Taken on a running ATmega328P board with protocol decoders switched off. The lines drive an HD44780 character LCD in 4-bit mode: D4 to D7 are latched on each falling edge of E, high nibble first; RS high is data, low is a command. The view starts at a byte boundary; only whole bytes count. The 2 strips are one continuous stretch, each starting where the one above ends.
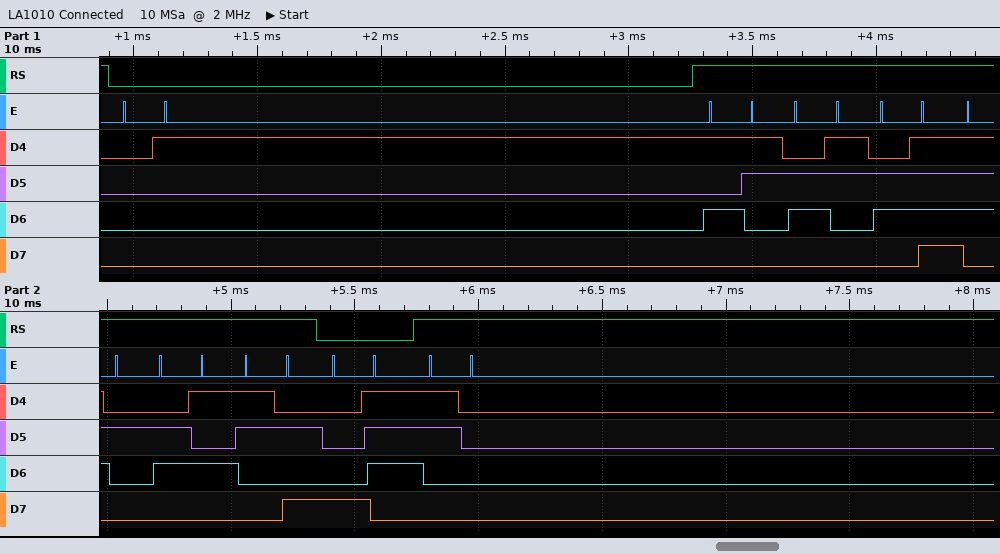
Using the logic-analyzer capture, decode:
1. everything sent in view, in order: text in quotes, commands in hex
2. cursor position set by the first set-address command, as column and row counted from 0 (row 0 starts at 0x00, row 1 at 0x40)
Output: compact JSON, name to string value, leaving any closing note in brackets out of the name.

{"everything sent in view, in order: text in quotes, commands in hex": "0x01 \"Score:\" 0x87 \"0\"", "cursor position set by the first set-address command, as column and row counted from 0": "column 7, row 0"}
